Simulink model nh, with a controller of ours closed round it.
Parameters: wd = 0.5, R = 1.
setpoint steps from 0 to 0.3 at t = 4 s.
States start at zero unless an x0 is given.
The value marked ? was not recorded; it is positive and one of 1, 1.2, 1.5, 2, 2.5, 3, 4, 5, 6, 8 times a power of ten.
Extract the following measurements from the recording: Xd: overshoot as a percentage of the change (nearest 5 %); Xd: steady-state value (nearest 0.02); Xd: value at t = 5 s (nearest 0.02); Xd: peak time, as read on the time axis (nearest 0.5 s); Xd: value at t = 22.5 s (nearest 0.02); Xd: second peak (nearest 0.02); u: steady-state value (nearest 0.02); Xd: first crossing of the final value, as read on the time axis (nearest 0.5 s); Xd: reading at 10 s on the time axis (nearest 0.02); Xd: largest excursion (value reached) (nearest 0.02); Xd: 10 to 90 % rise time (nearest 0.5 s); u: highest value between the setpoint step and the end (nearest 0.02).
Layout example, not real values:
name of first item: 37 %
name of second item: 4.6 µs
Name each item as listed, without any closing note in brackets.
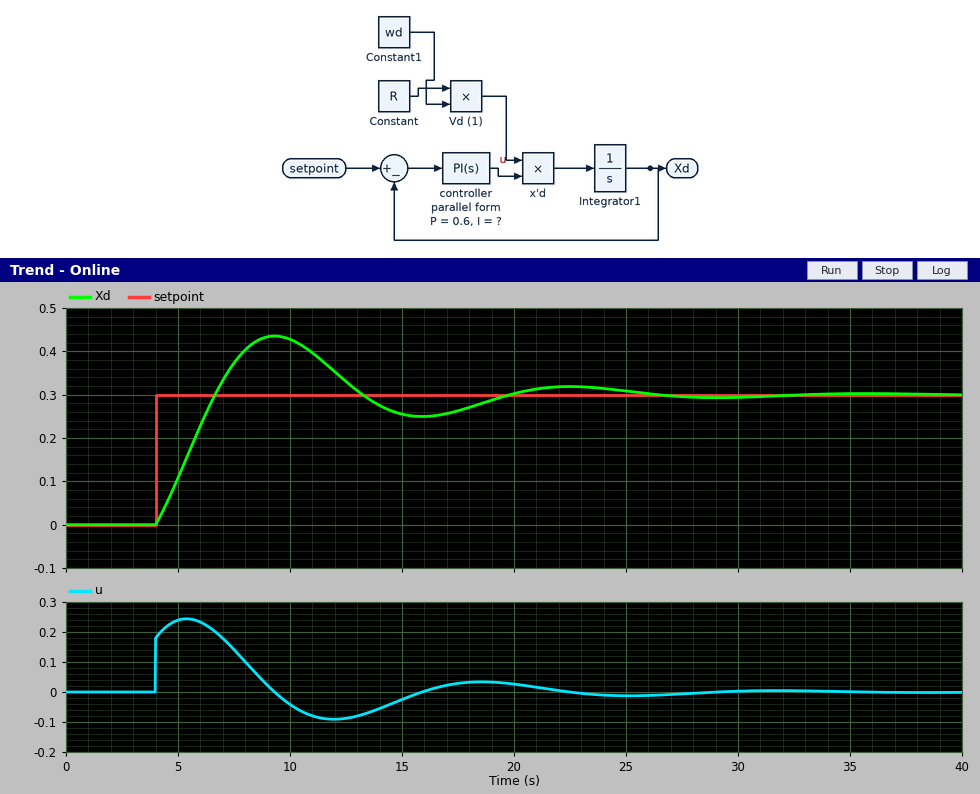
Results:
Xd: overshoot as a percentage of the change: 45 %
Xd: steady-state value: 0.30
Xd: value at t = 5 s: 0.10
Xd: peak time, as read on the time axis: 9.5 s
Xd: value at t = 22.5 s: 0.32
Xd: second peak: 0.32
u: steady-state value: 0.00
Xd: first crossing of the final value, as read on the time axis: 6.5 s
Xd: reading at 10 s on the time axis: 0.42
Xd: largest excursion (value reached): 0.44
Xd: 10 to 90 % rise time: 2.0 s
u: highest value between the setpoint step and the end: 0.24
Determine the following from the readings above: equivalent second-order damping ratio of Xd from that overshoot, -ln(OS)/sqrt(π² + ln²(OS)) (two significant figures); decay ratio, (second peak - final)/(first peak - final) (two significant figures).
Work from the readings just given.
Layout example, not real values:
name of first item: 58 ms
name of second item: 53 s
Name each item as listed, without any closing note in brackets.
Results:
equivalent second-order damping ratio of Xd from that overshoot, -ln(OS)/sqrt(π² + ln²(OS)): 0.25
decay ratio, (second peak - final)/(first peak - final): 0.14
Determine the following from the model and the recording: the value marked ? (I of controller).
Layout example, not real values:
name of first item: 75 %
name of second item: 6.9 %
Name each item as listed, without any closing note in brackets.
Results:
the value marked ?: 0.5
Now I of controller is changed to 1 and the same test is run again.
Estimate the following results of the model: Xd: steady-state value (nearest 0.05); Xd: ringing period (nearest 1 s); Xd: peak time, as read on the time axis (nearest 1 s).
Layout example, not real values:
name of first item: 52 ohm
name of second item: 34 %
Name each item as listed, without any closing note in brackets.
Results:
Xd: steady-state value: 0.30
Xd: ringing period: 9 s
Xd: peak time, as read on the time axis: 8 s
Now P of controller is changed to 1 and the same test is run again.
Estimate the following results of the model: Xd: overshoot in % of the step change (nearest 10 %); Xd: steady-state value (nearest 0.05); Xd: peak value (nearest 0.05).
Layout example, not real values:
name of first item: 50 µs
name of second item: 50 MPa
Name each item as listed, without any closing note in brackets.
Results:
Xd: overshoot in % of the step change: 30 %
Xd: steady-state value: 0.30
Xd: peak value: 0.40
